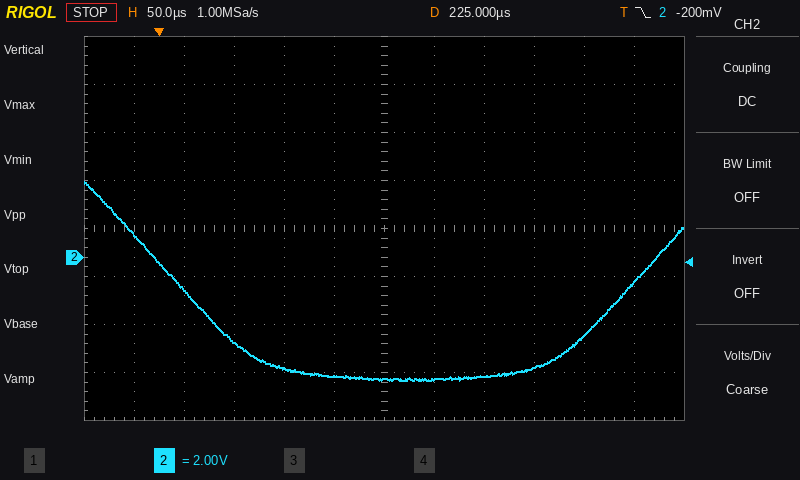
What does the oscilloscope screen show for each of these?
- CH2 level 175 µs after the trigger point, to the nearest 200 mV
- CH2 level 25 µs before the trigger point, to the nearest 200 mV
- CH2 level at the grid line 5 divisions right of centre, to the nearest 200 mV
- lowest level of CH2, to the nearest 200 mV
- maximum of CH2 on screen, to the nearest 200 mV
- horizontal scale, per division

-5.0 V
1.0 V
-1.0 V
-5.2 V
3.2 V
50 µs
